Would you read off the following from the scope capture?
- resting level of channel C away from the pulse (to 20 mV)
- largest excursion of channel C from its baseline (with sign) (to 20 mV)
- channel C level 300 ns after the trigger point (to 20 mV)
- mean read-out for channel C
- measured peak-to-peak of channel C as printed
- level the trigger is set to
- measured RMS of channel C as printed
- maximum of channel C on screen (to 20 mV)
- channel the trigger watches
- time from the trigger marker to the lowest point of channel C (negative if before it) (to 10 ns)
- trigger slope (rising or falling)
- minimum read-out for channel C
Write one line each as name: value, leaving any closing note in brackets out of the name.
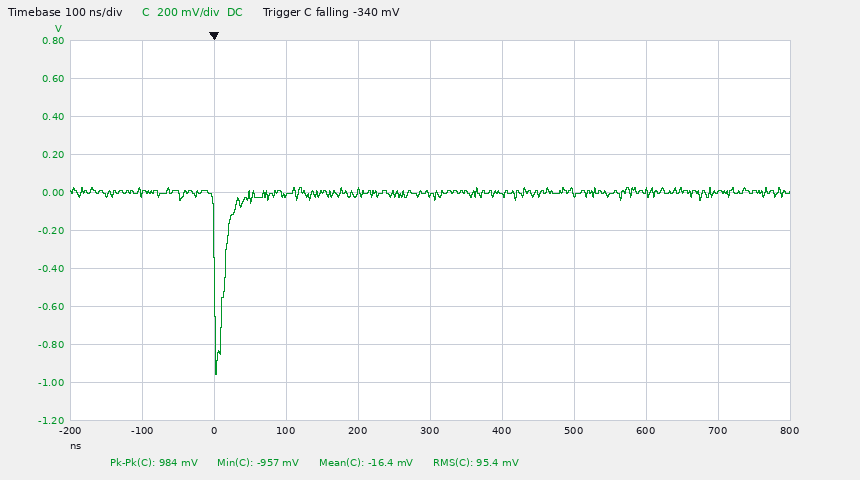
resting level of channel C away from the pulse: 0 mV
largest excursion of channel C from its baseline (with sign): -960 mV
channel C level 300 ns after the trigger point: 0 mV
mean read-out for channel C: -16.4 mV
measured peak-to-peak of channel C as printed: 984 mV
level the trigger is set to: -340 mV
measured RMS of channel C as printed: 95.4 mV
maximum of channel C on screen: 20 mV
channel the trigger watches: channel C
time from the trigger marker to the lowest point of channel C (negative if before it): 0 ns
trigger slope: falling
minimum read-out for channel C: -957 mV
